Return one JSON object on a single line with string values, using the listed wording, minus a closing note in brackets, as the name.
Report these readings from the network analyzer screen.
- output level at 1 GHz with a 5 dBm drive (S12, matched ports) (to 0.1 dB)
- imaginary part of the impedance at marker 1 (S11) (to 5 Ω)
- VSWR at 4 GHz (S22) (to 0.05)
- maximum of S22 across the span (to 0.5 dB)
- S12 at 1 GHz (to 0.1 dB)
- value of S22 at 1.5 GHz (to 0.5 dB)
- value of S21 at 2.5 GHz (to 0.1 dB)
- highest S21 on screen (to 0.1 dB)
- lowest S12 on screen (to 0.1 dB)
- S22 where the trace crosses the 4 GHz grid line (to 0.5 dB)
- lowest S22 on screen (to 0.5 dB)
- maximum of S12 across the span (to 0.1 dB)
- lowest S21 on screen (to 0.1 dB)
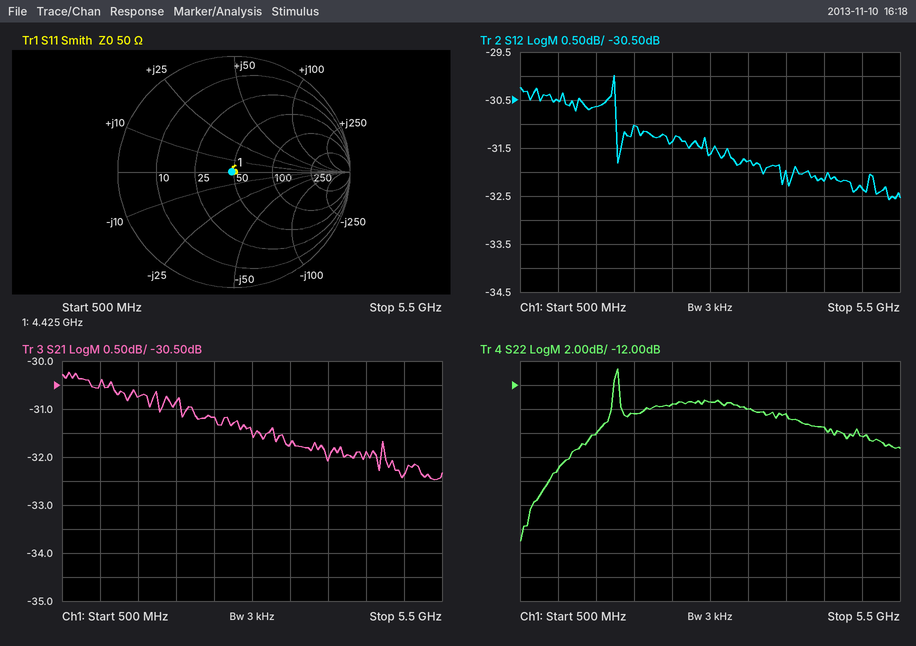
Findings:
{"output level at 1 GHz with a 5 dBm drive (S12, matched ports)": "-25.5 dBm", "imaginary part of the impedance at marker 1 (S11)": "0 Ω", "VSWR at 4 GHz (S22)": "1.45", "maximum of S22 across the span": "-10.5 dB", "S12 at 1 GHz": "-30.5 dB", "value of S22 at 1.5 GHz": "-16.0 dB", "value of S21 at 2.5 GHz": "-31.2 dB", "highest S21 on screen": "-30.2 dB", "lowest S12 on screen": "-32.6 dB", "S22 where the trace crosses the 4 GHz grid line": "-14.5 dB", "lowest S22 on screen": "-25.0 dB", "maximum of S12 across the span": "-30.0 dB", "lowest S21 on screen": "-32.5 dB"}
